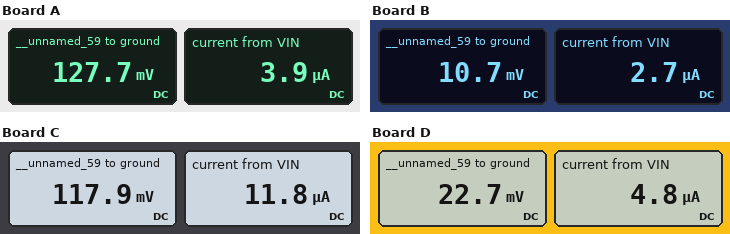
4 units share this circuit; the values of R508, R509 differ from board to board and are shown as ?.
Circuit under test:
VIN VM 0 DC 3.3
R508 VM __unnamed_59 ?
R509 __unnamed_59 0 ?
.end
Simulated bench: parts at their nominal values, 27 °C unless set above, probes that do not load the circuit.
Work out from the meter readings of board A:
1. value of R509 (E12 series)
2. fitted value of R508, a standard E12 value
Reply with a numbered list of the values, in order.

1. 33 kΩ
2. 820 kΩ
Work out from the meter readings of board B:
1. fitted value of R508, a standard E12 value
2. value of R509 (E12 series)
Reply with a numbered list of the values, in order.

1. 1.2 MΩ
2. 3.9 kΩ
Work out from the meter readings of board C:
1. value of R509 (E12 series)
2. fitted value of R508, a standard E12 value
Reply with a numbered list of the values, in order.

1. 10 kΩ
2. 270 kΩ
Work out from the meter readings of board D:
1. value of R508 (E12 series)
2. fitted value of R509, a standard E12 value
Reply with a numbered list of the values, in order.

1. 680 kΩ
2. 4.7 kΩ
